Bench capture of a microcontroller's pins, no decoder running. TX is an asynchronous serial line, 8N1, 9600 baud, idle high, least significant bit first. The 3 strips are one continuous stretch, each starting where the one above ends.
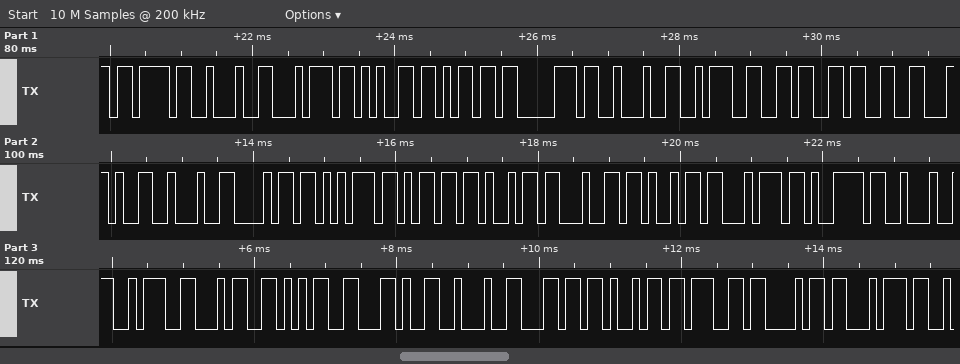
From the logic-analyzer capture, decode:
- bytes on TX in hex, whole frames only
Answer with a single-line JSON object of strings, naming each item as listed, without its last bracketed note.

{"bytes on TX in hex, whole frames only": "0x7B 0x22 0x74 0x65 0x6D 0x70 0x22 0x3A 0x36 0x33 0x2C 0x22 0x68 0x75 0x6D 0x69 0x64 0x69 0x74 0x79 0x22 0x3A 0x34 0x35 0x2C 0x22 0x6C 0x69 0x67 0x68 0x74"}
